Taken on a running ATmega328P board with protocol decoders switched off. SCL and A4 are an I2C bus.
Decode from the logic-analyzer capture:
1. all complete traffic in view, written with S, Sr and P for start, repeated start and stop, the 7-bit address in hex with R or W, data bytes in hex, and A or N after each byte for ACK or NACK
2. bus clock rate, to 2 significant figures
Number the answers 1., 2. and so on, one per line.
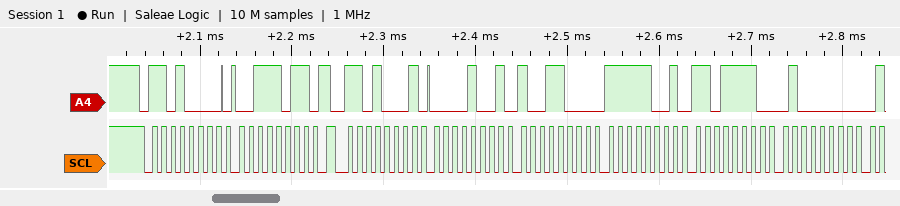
1. S 68W A 3B A Sr 68R A 09 A 98 A F9 A DE A 40 A
2. 100 kHz
